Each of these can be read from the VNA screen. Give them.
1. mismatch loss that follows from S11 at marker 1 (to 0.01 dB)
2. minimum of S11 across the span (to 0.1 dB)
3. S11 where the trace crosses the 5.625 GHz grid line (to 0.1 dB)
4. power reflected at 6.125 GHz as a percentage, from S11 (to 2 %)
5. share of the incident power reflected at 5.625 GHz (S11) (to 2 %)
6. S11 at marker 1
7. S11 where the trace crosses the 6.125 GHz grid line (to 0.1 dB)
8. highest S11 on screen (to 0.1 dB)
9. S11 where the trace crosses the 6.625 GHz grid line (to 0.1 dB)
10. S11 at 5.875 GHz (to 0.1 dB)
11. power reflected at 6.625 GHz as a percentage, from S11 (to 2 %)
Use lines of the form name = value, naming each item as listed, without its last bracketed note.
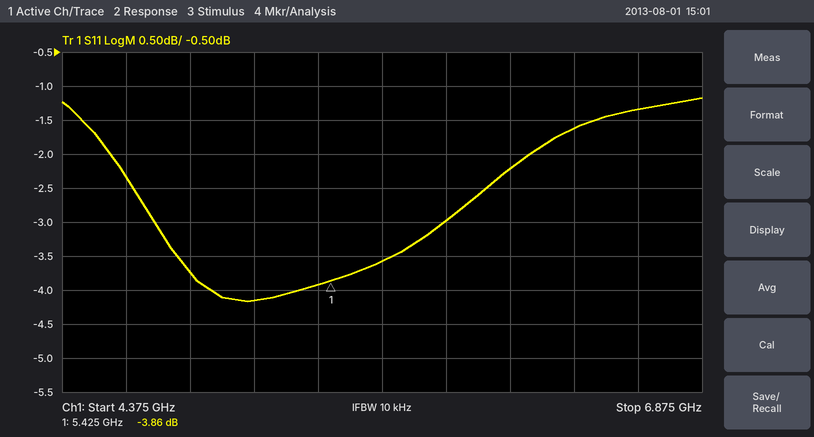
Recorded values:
mismatch loss that follows from S11 at marker 1 = 2.30 dB
minimum of S11 across the span = -4.2 dB
S11 where the trace crosses the 5.625 GHz grid line = -3.6 dB
power reflected at 6.125 GHz as a percentage, from S11 = 60 %
share of the incident power reflected at 5.625 GHz (S11) = 44 %
S11 at marker 1 = -3.86 dB
S11 where the trace crosses the 6.125 GHz grid line = -2.2 dB
highest S11 on screen = -1.2 dB
S11 where the trace crosses the 6.625 GHz grid line = -1.3 dB
S11 at 5.875 GHz = -3.0 dB
power reflected at 6.625 GHz as a percentage, from S11 = 74 %
